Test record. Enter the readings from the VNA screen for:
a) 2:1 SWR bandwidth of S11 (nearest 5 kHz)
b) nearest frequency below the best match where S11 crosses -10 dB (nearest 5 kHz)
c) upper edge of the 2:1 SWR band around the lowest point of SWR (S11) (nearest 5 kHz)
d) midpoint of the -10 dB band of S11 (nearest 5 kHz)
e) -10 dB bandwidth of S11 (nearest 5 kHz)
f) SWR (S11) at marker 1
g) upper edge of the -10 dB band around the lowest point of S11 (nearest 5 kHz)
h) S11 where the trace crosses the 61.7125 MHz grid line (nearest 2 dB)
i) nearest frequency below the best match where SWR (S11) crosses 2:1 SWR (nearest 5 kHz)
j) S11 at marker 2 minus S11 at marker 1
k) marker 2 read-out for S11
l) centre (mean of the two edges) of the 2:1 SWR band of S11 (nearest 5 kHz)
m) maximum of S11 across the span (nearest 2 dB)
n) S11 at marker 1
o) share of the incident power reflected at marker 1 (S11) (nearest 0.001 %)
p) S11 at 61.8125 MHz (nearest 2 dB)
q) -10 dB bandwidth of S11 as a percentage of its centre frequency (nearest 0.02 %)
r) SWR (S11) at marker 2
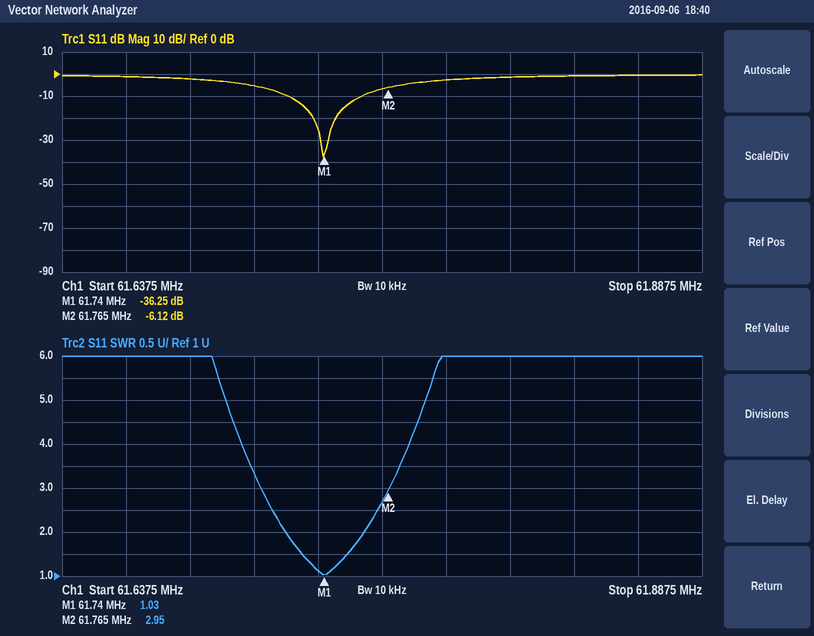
30 kHz
61.725 MHz
61.755 MHz
61.740 MHz
30 kHz
1.03
61.755 MHz
-6 dB
61.725 MHz
30.13 dB
-6.12 dB
61.740 MHz
0 dB
-36.25 dB
0.024 %
-2 dB
0.04 %
2.95
